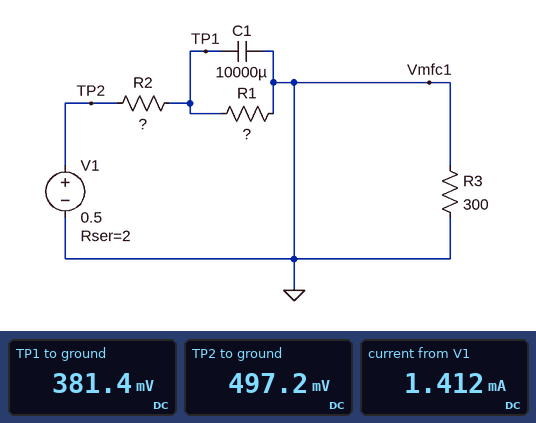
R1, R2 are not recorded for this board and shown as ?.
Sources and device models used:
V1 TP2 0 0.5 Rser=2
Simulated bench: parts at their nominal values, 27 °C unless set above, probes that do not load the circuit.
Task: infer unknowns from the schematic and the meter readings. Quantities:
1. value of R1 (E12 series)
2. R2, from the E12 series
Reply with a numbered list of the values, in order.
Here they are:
1. 270 Ω
2. 82 Ω
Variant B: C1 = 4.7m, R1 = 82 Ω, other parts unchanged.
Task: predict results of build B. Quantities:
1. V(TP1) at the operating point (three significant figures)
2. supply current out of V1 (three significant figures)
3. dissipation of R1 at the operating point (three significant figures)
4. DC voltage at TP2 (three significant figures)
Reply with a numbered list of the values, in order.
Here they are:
1. 247 mV
2. 3.01 mA
3. 744 µW
4. 494 mV
